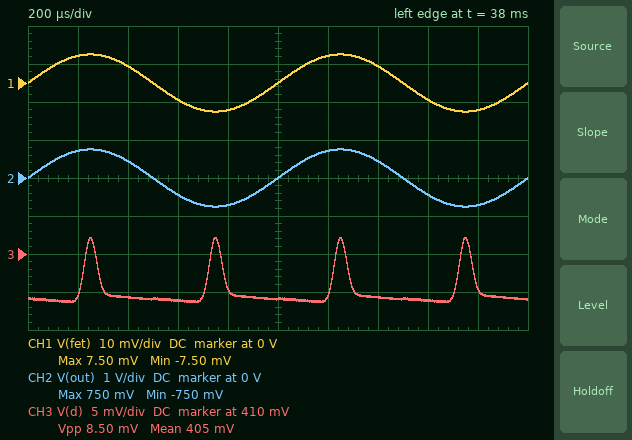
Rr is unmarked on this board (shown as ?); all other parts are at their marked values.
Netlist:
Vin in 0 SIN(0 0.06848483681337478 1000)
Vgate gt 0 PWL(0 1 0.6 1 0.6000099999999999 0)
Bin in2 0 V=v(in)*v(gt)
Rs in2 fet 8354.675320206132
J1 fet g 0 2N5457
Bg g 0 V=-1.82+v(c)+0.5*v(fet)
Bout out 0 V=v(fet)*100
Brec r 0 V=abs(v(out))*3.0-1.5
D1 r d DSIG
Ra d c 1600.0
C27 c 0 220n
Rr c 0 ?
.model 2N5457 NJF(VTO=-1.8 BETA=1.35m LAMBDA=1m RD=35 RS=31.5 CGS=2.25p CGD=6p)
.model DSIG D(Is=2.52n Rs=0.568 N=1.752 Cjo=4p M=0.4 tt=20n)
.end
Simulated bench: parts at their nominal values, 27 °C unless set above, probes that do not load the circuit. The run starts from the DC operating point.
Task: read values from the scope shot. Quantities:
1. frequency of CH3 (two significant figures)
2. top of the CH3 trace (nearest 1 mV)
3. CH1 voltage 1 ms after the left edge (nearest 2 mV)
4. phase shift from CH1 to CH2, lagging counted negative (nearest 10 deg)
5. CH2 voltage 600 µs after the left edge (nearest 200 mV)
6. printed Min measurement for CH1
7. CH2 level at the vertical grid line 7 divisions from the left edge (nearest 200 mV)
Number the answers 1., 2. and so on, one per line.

1. 2.0 kHz
2. 412 mV
3. 0 V
4. 0 deg
5. -400 mV
6. -7.50 mV
7. 400 mV
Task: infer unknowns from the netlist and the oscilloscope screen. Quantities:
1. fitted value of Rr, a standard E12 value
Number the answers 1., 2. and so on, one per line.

1. 680 kΩ
